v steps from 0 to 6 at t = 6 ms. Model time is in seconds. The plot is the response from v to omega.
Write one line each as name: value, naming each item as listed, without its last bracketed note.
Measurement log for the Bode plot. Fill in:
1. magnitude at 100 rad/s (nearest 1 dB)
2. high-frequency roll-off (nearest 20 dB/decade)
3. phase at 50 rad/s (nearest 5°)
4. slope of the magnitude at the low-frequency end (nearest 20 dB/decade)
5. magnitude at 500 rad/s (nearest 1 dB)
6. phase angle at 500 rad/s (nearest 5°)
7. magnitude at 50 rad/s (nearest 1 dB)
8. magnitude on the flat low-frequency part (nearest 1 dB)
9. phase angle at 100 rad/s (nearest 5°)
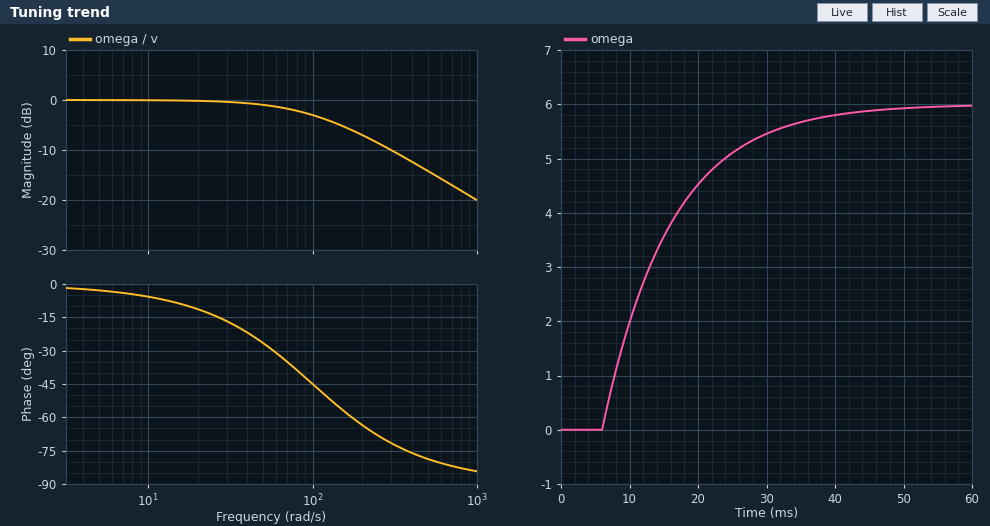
magnitude at 100 rad/s: -3 dB
high-frequency roll-off: -20 dB/decade
phase at 50 rad/s: -25°
slope of the magnitude at the low-frequency end: 0 dB/decade
magnitude at 500 rad/s: -14 dB
phase angle at 500 rad/s: -80°
magnitude at 50 rad/s: -1 dB
magnitude on the flat low-frequency part: 0 dB
phase angle at 100 rad/s: -45°
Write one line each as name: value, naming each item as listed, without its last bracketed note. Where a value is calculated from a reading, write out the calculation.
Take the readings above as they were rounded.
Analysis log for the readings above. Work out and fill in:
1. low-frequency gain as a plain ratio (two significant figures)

low-frequency gain as a plain ratio: 10^(0 / 20) = 1.0
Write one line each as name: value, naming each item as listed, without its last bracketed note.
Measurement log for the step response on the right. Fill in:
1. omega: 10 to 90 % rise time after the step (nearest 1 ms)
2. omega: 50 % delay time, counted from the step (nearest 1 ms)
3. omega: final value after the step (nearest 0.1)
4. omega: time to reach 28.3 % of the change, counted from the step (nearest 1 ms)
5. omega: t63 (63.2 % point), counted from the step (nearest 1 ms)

omega: 10 to 90 % rise time after the step: 22 ms
omega: 50 % delay time, counted from the step: 7 ms
omega: final value after the step: 6.0
omega: time to reach 28.3 % of the change, counted from the step: 3 ms
omega: t63 (63.2 % point), counted from the step: 10 ms
